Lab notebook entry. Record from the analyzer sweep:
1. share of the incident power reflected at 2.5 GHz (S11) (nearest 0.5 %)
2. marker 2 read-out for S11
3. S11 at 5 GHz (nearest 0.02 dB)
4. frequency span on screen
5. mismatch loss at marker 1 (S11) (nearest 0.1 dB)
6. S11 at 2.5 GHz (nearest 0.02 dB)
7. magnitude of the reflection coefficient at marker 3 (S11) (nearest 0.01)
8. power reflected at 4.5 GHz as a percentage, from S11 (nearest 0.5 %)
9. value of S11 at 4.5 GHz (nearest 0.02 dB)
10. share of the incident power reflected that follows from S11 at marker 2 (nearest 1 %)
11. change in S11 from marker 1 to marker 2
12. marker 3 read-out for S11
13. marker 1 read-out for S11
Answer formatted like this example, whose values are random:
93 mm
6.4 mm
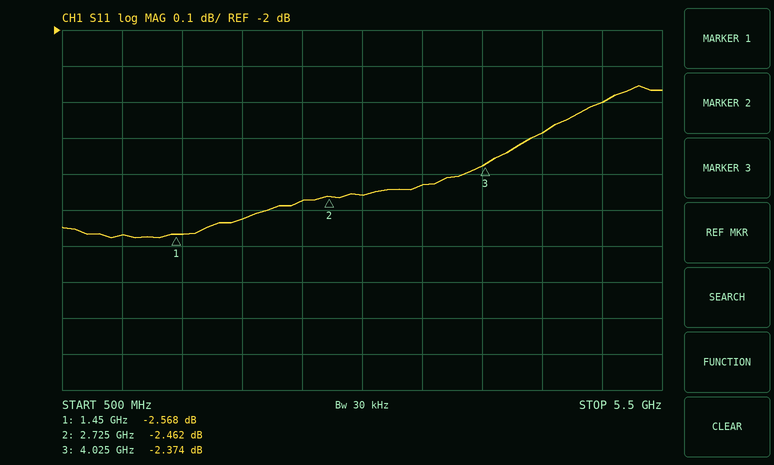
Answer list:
56.5 %
-2.462 dB
-2.20 dB
5 GHz
3.5 dB
-2.48 dB
0.76
59.0 %
-2.28 dB
57 %
0.106 dB
-2.374 dB
-2.568 dB
